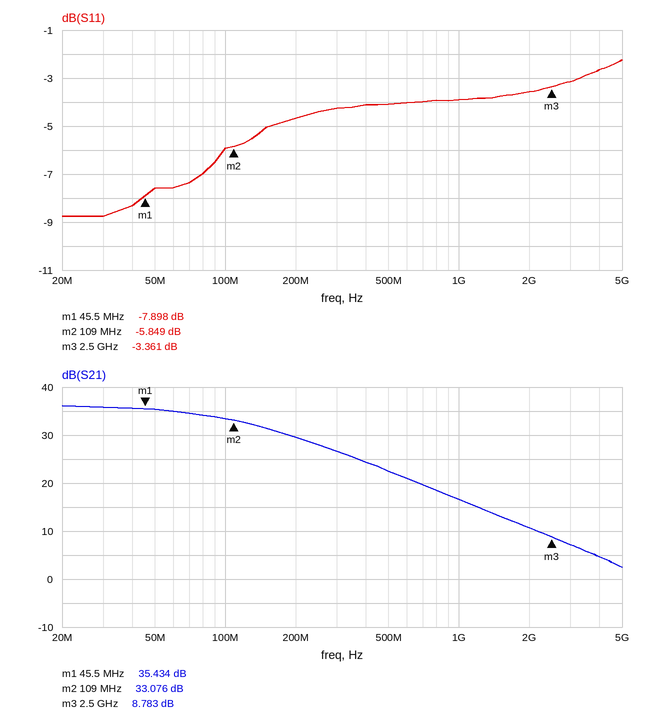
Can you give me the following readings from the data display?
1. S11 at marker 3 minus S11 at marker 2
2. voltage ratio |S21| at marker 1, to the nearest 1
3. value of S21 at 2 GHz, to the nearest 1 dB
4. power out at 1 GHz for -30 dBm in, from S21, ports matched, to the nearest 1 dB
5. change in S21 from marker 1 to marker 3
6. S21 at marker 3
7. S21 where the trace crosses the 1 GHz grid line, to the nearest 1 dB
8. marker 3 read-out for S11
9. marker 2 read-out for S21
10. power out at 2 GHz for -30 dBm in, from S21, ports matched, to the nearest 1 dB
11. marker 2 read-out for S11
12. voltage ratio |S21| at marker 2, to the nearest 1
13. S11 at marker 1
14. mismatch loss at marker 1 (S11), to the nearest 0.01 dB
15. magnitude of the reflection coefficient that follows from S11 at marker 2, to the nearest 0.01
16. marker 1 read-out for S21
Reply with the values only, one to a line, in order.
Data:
2.488 dB
59
11 dB
-13 dBm
-26.651 dB
8.783 dB
17 dB
-3.361 dB
33.076 dB
-19 dBm
-5.849 dB
45
-7.898 dB
0.77 dB
0.51
35.434 dB
